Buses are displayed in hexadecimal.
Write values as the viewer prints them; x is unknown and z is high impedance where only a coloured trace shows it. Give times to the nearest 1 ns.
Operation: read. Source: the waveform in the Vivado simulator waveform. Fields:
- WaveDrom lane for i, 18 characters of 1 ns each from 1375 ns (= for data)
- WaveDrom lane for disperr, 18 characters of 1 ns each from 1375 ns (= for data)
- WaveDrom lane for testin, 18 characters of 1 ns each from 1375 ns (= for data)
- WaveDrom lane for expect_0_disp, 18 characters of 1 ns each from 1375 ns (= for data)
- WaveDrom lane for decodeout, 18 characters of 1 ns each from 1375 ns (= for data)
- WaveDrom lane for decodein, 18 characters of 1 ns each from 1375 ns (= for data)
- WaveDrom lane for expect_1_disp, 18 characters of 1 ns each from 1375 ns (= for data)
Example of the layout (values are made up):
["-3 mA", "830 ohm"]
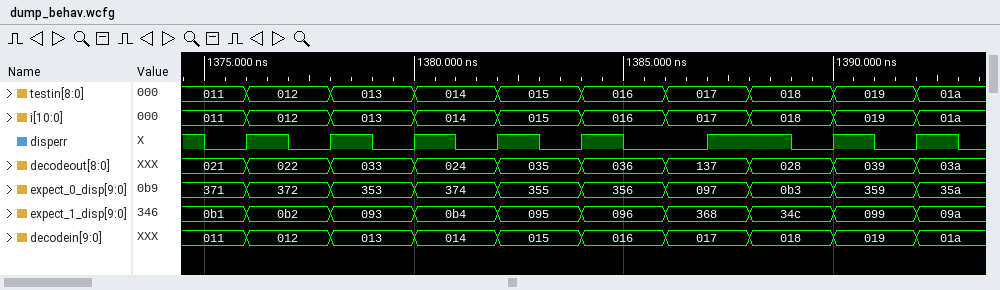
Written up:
["{name: 'i', wave: '==.=.=.=.=.=.=.=.=', data: '011 012 013 014 015 016 017 018 019 01a'}", "{name: 'disperr', wave: '01010101010.1.0101'}", "{name: 'testin', wave: '==.=.=.=.=.=.=.=.=', data: '011 012 013 014 015 016 017 018 019 01a'}", "{name: 'expect_0_disp', wave: '==.=.=.=.=.=.=.=.=', data: '371 372 353 374 355 356 097 0b3 359 35a'}", "{name: 'decodeout', wave: '==.=.=.=.=.=.=.=.=', data: '021 022 033 024 035 036 137 028 039 03a'}", "{name: 'decodein', wave: '==.=.=.=.=.=.=.=.=', data: '011 012 013 014 015 016 017 018 019 01a'}", "{name: 'expect_1_disp', wave: '==.=.=.=.=.=.=.=.=', data: '0b1 0b2 093 0b4 095 096 368 34c 099 09a'}"]
